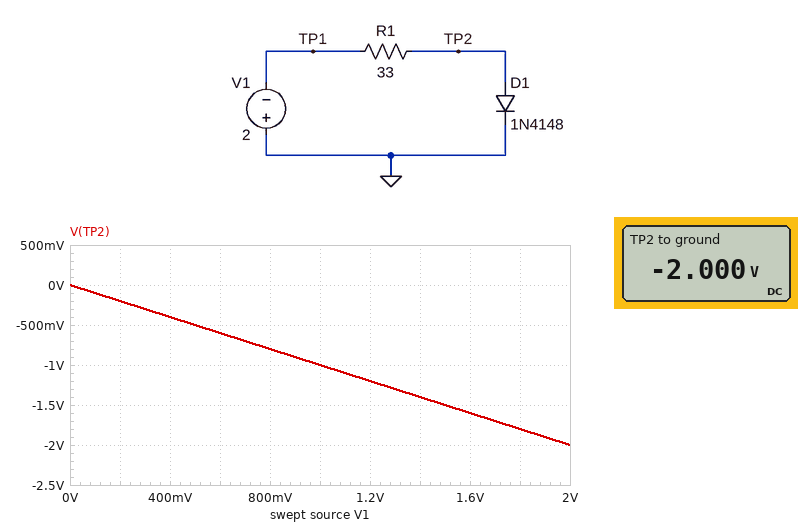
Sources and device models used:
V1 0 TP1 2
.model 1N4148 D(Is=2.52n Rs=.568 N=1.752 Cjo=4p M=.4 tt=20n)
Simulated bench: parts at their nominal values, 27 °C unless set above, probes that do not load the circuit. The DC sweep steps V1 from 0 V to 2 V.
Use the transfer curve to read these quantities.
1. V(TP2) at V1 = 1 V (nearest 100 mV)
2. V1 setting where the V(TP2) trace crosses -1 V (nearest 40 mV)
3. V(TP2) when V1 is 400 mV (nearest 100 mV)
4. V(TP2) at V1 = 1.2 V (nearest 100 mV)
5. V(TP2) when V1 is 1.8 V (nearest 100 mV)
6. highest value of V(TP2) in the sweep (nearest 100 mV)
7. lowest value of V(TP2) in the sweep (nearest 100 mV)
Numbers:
-1.0 V
1.00 V
-400 mV
-1.2 V
-1.8 V
0 V
-2.0 V
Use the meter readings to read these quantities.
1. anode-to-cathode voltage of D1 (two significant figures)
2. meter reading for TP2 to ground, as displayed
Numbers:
-2.0 V
-2.000 V
